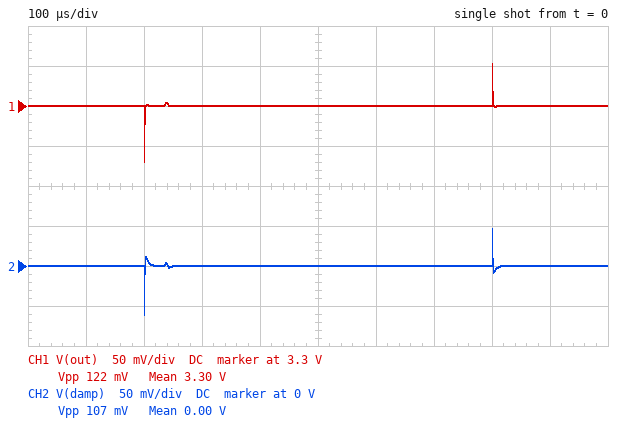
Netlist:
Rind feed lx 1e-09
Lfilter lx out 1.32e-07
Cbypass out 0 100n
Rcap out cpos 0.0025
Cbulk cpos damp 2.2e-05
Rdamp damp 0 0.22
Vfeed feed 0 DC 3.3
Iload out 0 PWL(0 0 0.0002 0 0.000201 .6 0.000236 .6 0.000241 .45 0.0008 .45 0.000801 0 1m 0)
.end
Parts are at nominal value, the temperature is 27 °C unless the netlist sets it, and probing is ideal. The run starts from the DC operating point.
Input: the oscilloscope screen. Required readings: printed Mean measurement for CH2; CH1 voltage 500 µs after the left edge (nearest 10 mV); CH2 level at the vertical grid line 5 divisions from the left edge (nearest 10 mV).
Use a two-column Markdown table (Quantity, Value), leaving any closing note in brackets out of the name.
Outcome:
| Quantity | Value |
|---|---|
| printed Mean measurement for CH2 | 0.00 V |
| CH1 voltage 500 µs after the left edge | 3.30 V |
| CH2 level at the vertical grid line 5 divisions from the left edge | 0 V |
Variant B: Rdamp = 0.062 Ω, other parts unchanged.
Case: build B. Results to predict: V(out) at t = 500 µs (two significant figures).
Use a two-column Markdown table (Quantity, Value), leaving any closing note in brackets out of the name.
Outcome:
| Quantity | Value |
|---|---|
| V(out) at t = 500 µs | 3.3 V |
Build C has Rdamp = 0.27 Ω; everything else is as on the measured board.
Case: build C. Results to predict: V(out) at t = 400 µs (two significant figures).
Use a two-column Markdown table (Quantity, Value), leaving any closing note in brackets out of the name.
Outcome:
| Quantity | Value |
|---|---|
| V(out) at t = 400 µs | 3.3 V |
